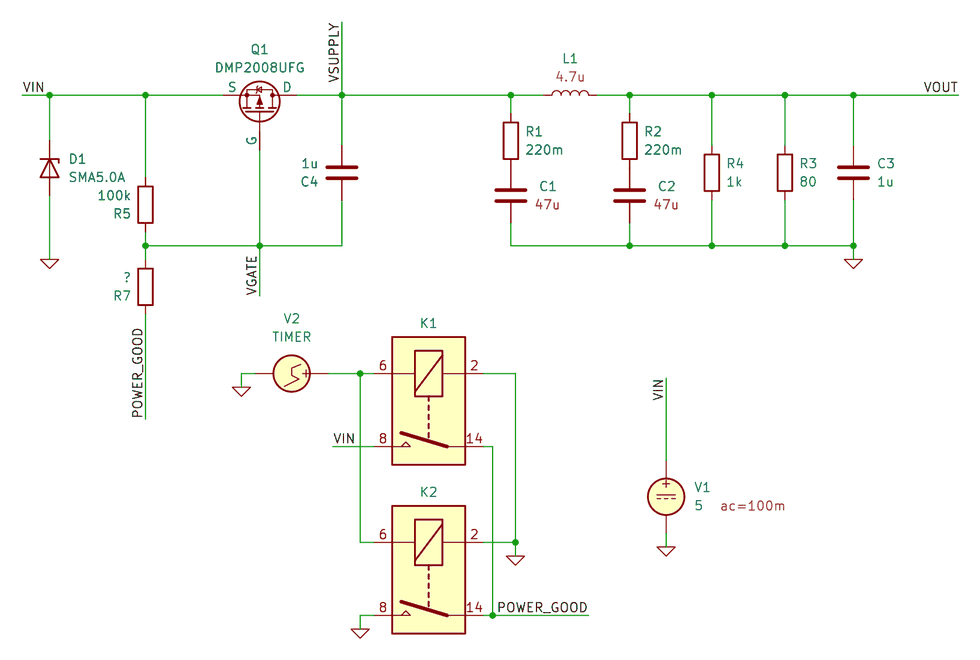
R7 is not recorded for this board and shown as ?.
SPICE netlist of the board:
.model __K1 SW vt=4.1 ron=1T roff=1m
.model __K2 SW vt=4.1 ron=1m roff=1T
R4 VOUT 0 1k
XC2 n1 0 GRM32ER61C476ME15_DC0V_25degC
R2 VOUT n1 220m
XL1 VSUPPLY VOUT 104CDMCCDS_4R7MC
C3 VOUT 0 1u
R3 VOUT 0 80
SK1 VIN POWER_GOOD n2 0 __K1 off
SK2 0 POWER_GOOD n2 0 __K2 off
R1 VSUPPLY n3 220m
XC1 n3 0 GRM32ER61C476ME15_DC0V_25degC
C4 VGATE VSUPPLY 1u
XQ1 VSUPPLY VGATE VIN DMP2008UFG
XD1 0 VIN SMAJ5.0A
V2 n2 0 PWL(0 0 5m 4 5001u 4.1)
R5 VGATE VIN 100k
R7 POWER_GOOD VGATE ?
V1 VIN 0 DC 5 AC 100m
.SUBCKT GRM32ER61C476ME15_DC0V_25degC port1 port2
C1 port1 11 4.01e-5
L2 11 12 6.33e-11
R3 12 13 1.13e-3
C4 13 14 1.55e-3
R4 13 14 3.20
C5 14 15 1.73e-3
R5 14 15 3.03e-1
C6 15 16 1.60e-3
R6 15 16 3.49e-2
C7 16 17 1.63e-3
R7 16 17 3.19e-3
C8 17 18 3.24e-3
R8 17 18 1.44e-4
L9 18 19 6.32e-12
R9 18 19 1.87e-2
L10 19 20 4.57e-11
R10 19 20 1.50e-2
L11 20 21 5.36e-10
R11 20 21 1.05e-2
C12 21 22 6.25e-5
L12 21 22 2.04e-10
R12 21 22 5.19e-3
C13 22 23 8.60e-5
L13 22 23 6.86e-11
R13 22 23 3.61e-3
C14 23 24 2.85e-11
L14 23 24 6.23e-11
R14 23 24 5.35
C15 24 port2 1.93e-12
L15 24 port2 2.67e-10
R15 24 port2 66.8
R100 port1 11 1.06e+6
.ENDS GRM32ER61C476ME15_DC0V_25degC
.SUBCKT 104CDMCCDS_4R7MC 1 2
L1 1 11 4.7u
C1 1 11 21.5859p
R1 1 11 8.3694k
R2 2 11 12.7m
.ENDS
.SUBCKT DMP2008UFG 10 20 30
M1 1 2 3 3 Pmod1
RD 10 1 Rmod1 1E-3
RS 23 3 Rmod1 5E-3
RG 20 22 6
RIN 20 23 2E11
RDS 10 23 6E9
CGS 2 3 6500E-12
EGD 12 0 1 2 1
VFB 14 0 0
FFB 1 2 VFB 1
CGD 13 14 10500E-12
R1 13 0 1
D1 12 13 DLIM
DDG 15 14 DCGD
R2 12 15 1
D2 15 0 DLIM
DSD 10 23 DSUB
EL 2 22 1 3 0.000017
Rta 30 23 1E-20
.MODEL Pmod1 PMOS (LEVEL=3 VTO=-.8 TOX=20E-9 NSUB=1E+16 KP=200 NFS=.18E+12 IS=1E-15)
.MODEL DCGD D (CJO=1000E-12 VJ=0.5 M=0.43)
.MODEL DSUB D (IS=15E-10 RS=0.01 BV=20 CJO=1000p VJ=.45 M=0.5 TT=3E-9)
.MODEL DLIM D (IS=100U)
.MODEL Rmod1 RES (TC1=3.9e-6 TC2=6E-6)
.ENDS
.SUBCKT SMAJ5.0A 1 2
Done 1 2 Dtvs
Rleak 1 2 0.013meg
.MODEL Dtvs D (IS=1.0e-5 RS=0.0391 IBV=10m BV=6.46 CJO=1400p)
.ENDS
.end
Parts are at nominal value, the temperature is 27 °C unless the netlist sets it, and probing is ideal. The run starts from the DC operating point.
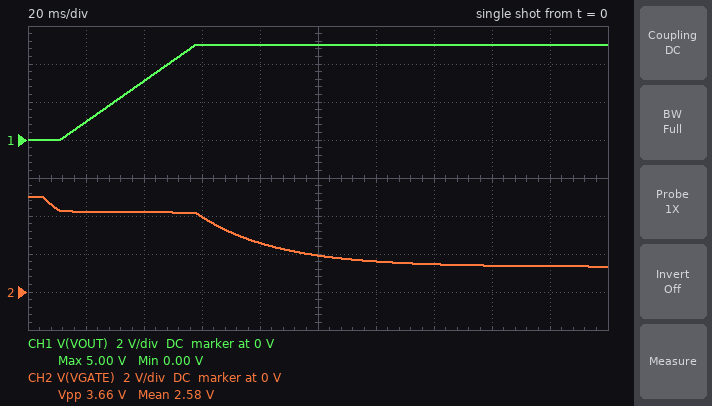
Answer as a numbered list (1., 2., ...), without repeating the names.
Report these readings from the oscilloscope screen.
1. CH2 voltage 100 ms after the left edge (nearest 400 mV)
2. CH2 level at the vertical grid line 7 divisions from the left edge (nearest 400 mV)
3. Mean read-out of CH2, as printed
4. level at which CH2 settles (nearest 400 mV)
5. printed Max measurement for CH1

1. 2.0 V
2. 1.6 V
3. 2.58 V
4. 1.2 V
5. 5.00 V
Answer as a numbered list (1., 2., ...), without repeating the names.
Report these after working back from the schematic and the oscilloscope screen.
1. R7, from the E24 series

1. 36 kΩ
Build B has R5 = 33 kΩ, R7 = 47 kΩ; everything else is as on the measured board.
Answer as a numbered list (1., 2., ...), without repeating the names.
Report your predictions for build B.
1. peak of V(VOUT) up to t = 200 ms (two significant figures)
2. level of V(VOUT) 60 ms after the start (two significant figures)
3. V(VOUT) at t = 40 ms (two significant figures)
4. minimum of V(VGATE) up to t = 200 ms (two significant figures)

1. 5.0 V
2. 3.0 V
3. 1.7 V
4. 2.9 V
